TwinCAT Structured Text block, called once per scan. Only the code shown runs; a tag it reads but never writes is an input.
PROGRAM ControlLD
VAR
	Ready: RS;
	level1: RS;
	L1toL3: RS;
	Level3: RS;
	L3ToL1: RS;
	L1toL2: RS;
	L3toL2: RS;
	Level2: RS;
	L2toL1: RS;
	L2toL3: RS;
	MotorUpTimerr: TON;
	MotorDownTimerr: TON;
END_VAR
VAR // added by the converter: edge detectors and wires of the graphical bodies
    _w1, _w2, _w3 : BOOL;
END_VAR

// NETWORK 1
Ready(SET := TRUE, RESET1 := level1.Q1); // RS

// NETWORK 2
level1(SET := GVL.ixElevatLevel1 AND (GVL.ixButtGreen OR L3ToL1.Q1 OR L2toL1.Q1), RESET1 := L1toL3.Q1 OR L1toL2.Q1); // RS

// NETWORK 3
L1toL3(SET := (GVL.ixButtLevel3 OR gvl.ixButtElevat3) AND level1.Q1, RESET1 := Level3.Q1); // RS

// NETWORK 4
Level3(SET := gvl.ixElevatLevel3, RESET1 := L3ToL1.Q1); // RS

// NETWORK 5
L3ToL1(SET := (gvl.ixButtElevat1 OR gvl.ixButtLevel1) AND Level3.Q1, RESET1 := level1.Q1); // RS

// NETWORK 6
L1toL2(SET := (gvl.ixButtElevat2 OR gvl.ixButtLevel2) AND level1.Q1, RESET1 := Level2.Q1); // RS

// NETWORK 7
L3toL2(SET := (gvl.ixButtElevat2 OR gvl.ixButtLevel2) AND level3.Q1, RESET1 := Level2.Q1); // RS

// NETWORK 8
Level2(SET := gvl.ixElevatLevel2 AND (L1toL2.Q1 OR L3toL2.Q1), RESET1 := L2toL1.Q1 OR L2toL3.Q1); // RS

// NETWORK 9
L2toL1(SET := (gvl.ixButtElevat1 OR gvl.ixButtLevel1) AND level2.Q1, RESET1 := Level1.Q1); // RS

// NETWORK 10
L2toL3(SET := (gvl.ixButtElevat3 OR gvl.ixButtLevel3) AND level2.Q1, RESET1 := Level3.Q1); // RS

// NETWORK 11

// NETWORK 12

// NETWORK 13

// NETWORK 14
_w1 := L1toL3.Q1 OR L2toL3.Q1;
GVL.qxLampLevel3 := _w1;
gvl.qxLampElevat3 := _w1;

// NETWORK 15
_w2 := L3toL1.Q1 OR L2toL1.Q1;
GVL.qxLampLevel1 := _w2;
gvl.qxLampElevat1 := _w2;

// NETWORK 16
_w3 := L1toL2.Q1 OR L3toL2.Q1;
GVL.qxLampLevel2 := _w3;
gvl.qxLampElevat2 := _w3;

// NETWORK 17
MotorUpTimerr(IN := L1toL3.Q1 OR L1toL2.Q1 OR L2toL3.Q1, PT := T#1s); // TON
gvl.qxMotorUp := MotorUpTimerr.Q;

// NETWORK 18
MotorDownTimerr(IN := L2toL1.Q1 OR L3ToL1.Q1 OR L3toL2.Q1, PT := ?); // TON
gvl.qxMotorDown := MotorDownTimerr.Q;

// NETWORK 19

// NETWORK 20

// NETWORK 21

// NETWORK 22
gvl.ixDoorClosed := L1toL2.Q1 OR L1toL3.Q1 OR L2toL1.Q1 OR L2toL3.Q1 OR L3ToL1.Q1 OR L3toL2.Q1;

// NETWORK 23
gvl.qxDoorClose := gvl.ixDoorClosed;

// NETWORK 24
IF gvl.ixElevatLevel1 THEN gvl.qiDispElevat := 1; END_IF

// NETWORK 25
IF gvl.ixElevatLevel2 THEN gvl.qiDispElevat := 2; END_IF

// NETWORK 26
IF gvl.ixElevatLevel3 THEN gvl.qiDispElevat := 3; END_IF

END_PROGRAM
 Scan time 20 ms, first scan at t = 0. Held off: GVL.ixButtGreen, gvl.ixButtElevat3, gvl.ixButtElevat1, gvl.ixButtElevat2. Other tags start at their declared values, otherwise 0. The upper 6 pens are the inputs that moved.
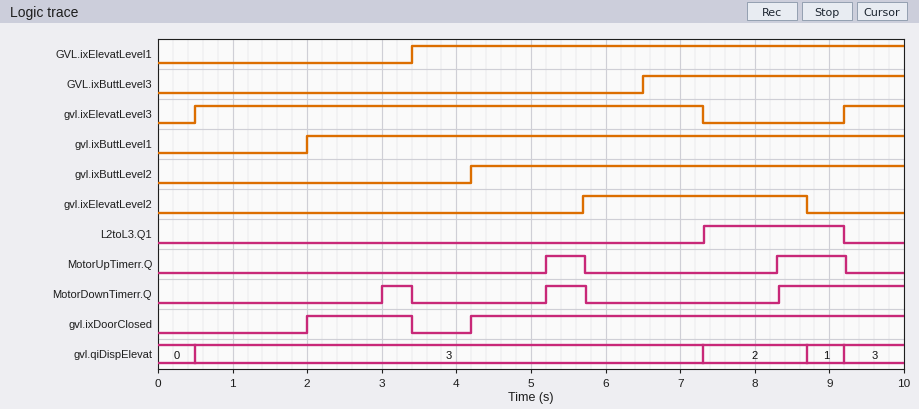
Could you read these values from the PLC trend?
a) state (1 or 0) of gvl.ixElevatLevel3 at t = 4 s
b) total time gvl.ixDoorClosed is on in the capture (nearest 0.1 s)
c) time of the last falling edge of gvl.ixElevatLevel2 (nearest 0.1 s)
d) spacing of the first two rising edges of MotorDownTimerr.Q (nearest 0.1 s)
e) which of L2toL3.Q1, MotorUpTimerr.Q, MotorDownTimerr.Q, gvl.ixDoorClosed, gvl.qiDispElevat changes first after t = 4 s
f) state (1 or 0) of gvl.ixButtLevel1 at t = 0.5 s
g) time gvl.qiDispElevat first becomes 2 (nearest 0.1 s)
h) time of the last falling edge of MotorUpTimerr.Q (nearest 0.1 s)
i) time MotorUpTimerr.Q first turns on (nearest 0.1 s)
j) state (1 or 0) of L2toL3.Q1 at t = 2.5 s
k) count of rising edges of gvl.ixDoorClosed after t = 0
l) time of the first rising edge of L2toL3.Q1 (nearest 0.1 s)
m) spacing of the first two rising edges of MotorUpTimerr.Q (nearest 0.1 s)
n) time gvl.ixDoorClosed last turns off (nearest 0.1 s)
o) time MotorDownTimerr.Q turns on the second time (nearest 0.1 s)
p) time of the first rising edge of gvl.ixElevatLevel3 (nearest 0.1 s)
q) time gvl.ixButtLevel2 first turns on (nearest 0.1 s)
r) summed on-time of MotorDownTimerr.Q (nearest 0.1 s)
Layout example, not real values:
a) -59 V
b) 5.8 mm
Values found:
a) 1
b) 7.2 s
c) 8.7 s
d) 2.2 s
e) gvl.ixDoorClosed
f) 0
g) 7.3 s
h) 9.2 s
i) 5.2 s
j) 0
k) 2
l) 7.3 s
m) 3.1 s
n) 3.4 s
o) 5.2 s
p) 0.5 s
q) 4.2 s
r) 2.6 s
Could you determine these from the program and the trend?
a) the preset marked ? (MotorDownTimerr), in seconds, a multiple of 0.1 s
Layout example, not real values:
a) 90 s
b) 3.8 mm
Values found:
a) 1.0 s
